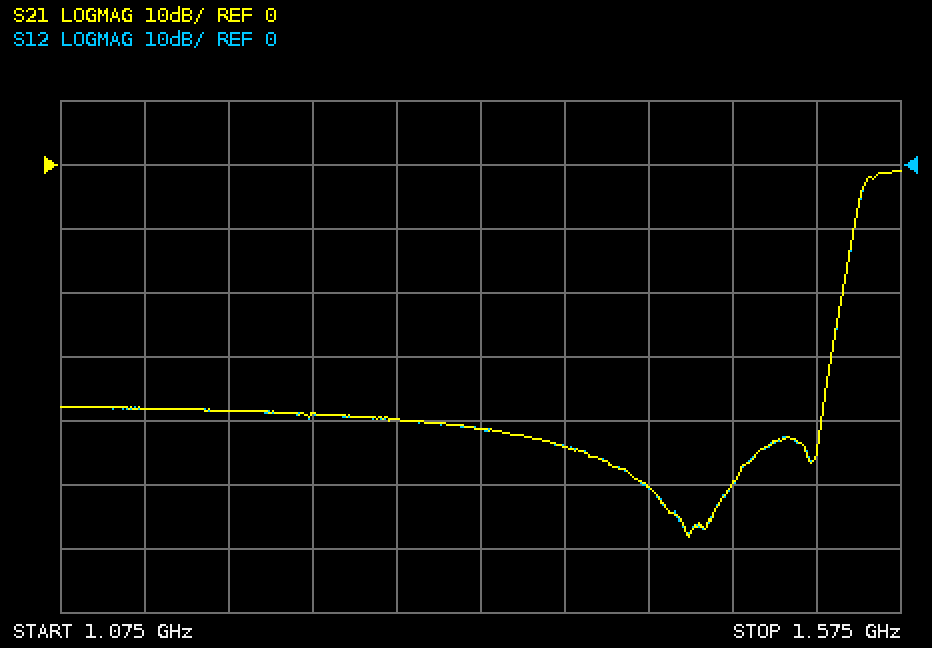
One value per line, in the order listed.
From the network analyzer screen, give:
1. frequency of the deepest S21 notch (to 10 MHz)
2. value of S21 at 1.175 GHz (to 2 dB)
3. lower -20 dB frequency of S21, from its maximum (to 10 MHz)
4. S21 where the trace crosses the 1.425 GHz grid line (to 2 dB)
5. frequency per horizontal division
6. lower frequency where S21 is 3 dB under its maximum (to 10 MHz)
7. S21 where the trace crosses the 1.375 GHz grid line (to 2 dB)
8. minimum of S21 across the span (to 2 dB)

1.45 GHz
-38 dB
1.54 GHz
-50 dB
50 MHz
1.55 GHz
-44 dB
-58 dB
